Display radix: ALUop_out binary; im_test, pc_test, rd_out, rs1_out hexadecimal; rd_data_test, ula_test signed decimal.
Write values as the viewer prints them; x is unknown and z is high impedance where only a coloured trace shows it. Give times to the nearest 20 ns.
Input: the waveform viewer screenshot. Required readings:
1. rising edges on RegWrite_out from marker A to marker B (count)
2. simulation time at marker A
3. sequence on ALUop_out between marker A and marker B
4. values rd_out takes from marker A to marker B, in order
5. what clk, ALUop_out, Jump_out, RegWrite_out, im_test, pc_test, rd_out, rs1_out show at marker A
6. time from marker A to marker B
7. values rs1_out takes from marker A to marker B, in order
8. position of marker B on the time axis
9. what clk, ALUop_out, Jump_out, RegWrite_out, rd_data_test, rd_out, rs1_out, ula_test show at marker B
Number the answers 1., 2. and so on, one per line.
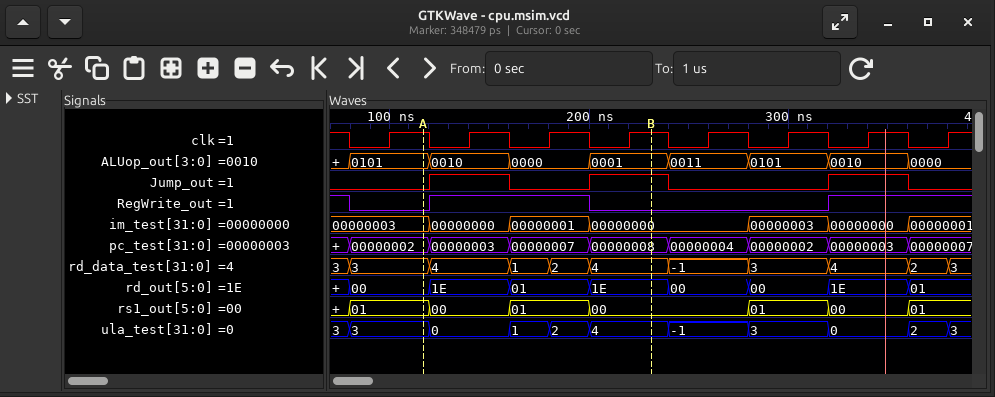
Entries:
1. 1
2. 120 ns
3. 0101, 0010, 0000, 0001
4. 00, 1E, 01, 1E
5. clk=1, ALUop_out=0101, Jump_out=0, RegWrite_out=0, im_test=00000003, pc_test=00000002, rd_out=00, rs1_out=01
6. 120 ns
7. 01, 00, 01, 00
8. 240 ns
9. clk=1, ALUop_out=0001, Jump_out=1, RegWrite_out=0, rd_data_test=4, rd_out=1E, rs1_out=00, ula_test=4
